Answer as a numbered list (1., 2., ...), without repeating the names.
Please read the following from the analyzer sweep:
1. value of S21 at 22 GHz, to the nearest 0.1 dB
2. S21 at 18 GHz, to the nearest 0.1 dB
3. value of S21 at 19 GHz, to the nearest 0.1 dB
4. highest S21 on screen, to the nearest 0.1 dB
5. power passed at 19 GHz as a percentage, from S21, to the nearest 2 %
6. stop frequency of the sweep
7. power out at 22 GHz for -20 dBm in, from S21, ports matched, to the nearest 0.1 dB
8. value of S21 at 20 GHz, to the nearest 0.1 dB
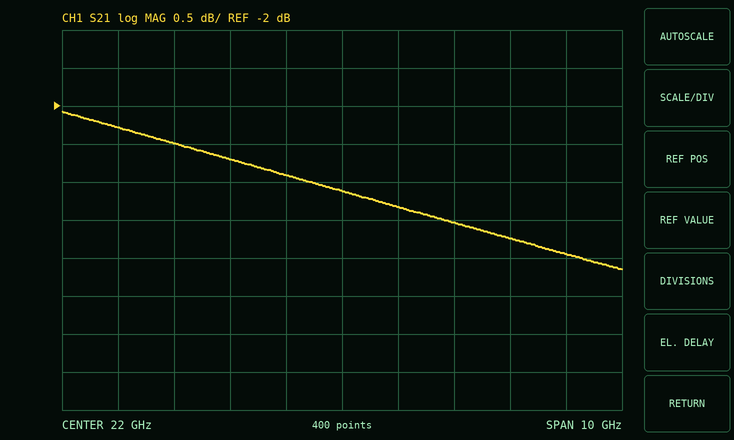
1. -3.1 dB
2. -2.3 dB
3. -2.5 dB
4. -2.1 dB
5. 56 %
6. 27 GHz
7. -23.1 dBm
8. -2.7 dB
